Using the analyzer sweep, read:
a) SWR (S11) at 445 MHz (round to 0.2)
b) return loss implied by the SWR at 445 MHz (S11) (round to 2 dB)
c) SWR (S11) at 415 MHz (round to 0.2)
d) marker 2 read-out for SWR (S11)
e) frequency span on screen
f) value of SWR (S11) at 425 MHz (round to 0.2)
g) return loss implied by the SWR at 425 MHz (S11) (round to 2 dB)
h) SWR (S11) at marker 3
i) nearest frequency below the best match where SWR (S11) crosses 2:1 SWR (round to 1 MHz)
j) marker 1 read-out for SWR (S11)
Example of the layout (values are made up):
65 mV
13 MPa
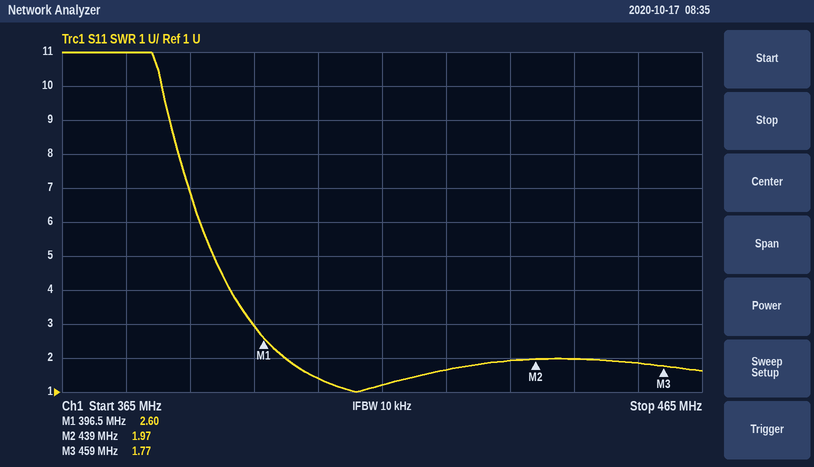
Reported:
2.0
10 dB
1.2
1.97
100 MHz
1.6
12 dB
1.77
400 MHz
2.60
